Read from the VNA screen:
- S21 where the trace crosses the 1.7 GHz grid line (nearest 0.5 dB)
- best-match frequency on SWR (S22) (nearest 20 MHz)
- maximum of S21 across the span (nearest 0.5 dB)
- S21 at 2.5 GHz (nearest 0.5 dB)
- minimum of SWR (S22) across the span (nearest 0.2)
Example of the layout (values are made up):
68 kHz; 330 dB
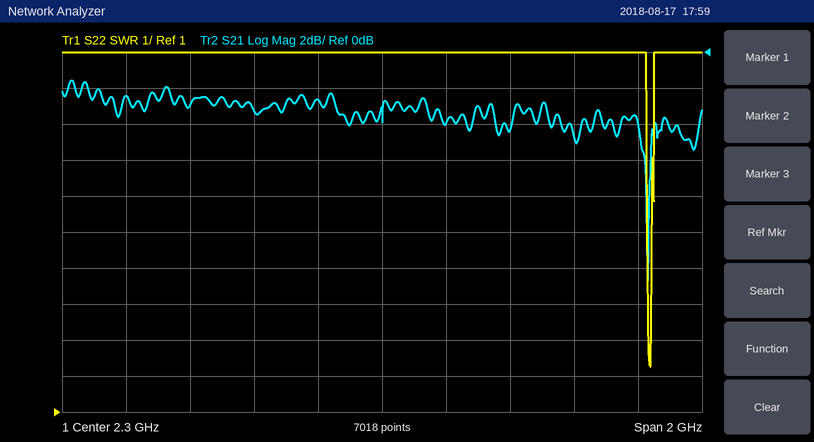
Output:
-3.0 dB; 3.14 GHz; -1.5 dB; -4.0 dB; 2.2
